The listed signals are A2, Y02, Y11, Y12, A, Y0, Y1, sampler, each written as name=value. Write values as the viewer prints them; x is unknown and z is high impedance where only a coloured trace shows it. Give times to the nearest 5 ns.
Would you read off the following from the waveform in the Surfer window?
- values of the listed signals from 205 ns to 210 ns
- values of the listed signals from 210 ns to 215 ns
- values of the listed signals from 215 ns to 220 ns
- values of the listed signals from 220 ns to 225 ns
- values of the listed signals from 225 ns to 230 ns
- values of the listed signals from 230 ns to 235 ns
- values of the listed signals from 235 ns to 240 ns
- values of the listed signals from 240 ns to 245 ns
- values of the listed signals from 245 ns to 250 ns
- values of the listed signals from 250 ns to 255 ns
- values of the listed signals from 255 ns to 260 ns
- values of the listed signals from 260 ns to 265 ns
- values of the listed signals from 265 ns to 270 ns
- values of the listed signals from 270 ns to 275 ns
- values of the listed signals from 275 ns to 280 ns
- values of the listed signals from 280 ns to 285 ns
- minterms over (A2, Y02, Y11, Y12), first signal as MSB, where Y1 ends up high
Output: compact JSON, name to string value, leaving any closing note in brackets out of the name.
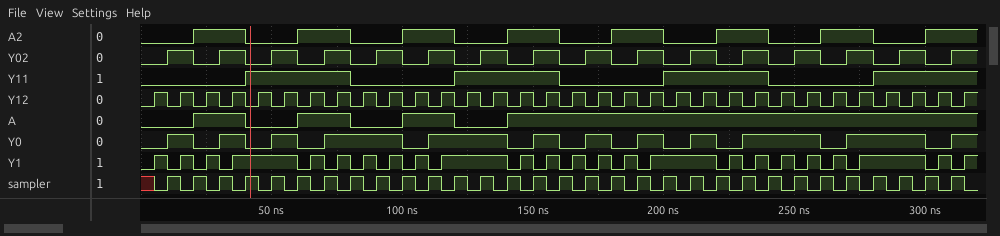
{"values of the listed signals from 205 ns to 210 ns": "A2=0, Y02=0, Y11=1, Y12=1, A=1, Y0=0, Y1=1, sampler=0", "values of the listed signals from 210 ns to 215 ns": "A2=0, Y02=1, Y11=1, Y12=0, A=1, Y0=1, Y1=1, sampler=1", "values of the listed signals from 215 ns to 220 ns": "A2=0, Y02=1, Y11=1, Y12=1, A=1, Y0=1, Y1=1, sampler=0", "values of the listed signals from 220 ns to 225 ns": "A2=1, Y02=0, Y11=1, Y12=0, A=1, Y0=0, Y1=0, sampler=1", "values of the listed signals from 225 ns to 230 ns": "A2=1, Y02=0, Y11=1, Y12=1, A=1, Y0=0, Y1=1, sampler=0", "values of the listed signals from 230 ns to 235 ns": "A2=1, Y02=1, Y11=1, Y12=0, A=1, Y0=1, Y1=0, sampler=1", "values of the listed signals from 235 ns to 240 ns": "A2=1, Y02=1, Y11=1, Y12=1, A=1, Y0=1, Y1=1, sampler=0", "values of the listed signals from 240 ns to 245 ns": "A2=0, Y02=0, Y11=0, Y12=0, A=1, Y0=1, Y1=0, sampler=1", "values of the listed signals from 245 ns to 250 ns": "A2=0, Y02=0, Y11=0, Y12=1, A=1, Y0=1, Y1=1, sampler=0", "values of the listed signals from 250 ns to 255 ns": "A2=0, Y02=1, Y11=0, Y12=0, A=1, Y0=1, Y1=0, sampler=1", "values of the listed signals from 255 ns to 260 ns": "A2=0, Y02=1, Y11=0, Y12=1, A=1, Y0=1, Y1=1, sampler=0", "values of the listed signals from 260 ns to 265 ns": "A2=1, Y02=0, Y11=0, Y12=0, A=1, Y0=0, Y1=0, sampler=1", "values of the listed signals from 265 ns to 270 ns": "A2=1, Y02=0, Y11=0, Y12=1, A=1, Y0=0, Y1=1, sampler=0", "values of the listed signals from 270 ns to 275 ns": "A2=1, Y02=1, Y11=0, Y12=0, A=1, Y0=1, Y1=0, sampler=1", "values of the listed signals from 275 ns to 280 ns": "A2=1, Y02=1, Y11=0, Y12=1, A=1, Y0=1, Y1=1, sampler=0", "values of the listed signals from 280 ns to 285 ns": "A2=0, Y02=0, Y11=1, Y12=0, A=1, Y0=1, Y1=1, sampler=1", "minterms over (A2, Y02, Y11, Y12), first signal as MSB, where Y1 ends up high": "1, 2, 3, 5, 6, 7, 9, 11, 13, 15"}
